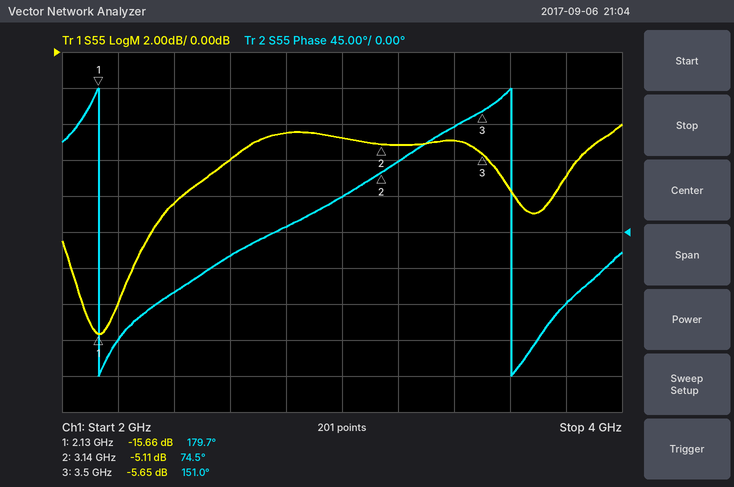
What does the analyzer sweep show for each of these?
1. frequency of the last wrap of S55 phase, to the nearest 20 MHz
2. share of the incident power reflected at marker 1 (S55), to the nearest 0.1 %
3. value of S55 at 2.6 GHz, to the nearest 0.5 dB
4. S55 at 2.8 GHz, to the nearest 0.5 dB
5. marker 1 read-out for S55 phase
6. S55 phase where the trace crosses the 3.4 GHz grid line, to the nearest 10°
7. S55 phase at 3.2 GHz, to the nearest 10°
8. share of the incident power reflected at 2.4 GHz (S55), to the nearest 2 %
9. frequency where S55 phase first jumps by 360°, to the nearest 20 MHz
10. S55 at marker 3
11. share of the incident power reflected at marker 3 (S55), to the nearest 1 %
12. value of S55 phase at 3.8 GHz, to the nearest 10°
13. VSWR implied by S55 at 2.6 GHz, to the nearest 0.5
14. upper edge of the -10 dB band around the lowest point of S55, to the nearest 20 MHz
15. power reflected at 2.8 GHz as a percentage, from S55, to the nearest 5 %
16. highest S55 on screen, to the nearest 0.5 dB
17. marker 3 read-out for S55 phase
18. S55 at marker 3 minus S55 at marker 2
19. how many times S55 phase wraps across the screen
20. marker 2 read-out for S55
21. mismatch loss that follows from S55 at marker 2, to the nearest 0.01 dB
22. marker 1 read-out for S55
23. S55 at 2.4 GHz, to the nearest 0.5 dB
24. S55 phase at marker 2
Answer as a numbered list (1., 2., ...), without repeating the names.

1. 3.60 GHz
2. 2.7 %
3. -6.0 dB
4. -4.5 dB
5. 179.7°
6. 130°
7. 90°
8. 14 %
9. 2.14 GHz
10. -5.65 dB
11. 27 %
12. -90°
13. 3.0
14. 2.32 GHz
15. 35 %
16. -4.0 dB
17. 151.0°
18. -0.54 dB
19. 2
20. -5.11 dB
21. 1.60 dB
22. -15.66 dB
23. -8.5 dB
24. 74.5°
